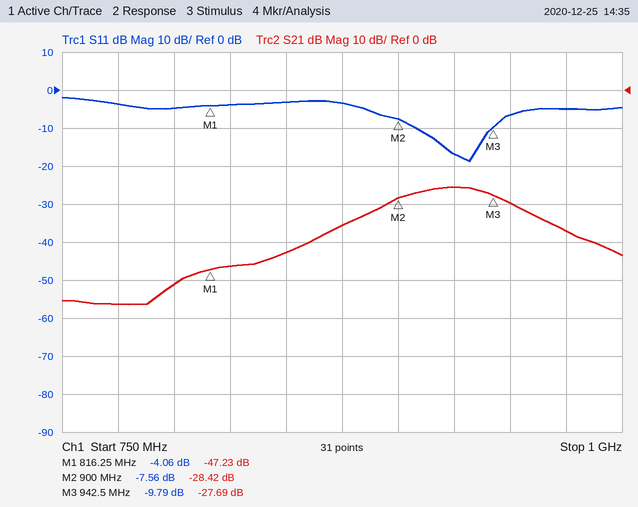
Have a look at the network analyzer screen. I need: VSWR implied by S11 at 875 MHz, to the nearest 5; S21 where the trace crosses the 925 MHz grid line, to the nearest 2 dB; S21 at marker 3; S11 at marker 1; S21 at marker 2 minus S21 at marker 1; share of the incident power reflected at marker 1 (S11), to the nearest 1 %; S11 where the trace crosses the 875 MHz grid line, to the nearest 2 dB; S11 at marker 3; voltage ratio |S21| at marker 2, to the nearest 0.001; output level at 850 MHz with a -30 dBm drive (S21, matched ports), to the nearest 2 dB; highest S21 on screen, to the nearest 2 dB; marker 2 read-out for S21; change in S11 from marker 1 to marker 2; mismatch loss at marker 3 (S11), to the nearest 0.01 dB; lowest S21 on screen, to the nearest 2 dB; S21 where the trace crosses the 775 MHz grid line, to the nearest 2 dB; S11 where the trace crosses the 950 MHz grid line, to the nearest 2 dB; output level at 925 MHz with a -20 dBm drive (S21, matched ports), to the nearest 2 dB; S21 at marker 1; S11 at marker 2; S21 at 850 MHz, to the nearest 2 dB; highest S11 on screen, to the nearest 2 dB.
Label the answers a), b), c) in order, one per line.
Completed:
a) 5
b) -26 dB
c) -27.69 dB
d) -4.06 dB
e) 18.81 dB
f) 39 %
g) -4 dB
h) -9.79 dB
i) 0.038
j) -72 dBm
k) -26 dB
l) -28.42 dB
m) -3.50 dB
n) 0.48 dB
o) -56 dB
p) -56 dB
q) -6 dB
r) -46 dBm
s) -47.23 dB
t) -7.56 dB
u) -42 dB
v) -2 dB
